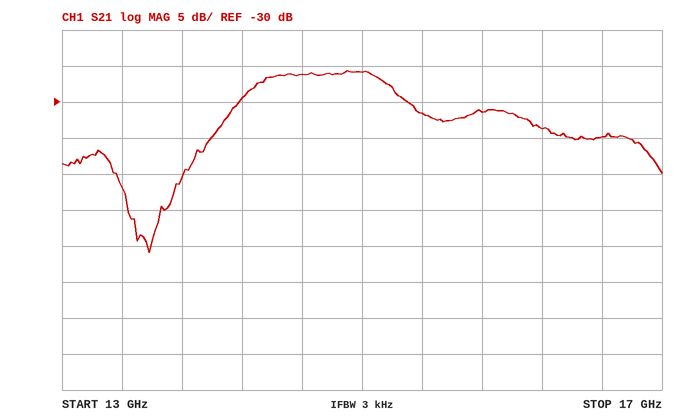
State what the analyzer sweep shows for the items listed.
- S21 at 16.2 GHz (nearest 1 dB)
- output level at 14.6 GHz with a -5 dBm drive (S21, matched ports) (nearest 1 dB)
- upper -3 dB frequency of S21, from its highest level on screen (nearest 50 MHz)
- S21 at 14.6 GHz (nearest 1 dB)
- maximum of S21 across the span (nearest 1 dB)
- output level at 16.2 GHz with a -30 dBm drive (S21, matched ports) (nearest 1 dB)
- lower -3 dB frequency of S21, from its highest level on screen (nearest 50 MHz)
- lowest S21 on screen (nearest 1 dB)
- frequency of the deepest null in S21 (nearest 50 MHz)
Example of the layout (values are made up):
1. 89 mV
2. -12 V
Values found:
1. -34 dB
2. -31 dBm
3. 15.20 GHz
4. -26 dB
5. -26 dB
6. -64 dBm
7. 14.25 GHz
8. -51 dB
9. 13.60 GHz
